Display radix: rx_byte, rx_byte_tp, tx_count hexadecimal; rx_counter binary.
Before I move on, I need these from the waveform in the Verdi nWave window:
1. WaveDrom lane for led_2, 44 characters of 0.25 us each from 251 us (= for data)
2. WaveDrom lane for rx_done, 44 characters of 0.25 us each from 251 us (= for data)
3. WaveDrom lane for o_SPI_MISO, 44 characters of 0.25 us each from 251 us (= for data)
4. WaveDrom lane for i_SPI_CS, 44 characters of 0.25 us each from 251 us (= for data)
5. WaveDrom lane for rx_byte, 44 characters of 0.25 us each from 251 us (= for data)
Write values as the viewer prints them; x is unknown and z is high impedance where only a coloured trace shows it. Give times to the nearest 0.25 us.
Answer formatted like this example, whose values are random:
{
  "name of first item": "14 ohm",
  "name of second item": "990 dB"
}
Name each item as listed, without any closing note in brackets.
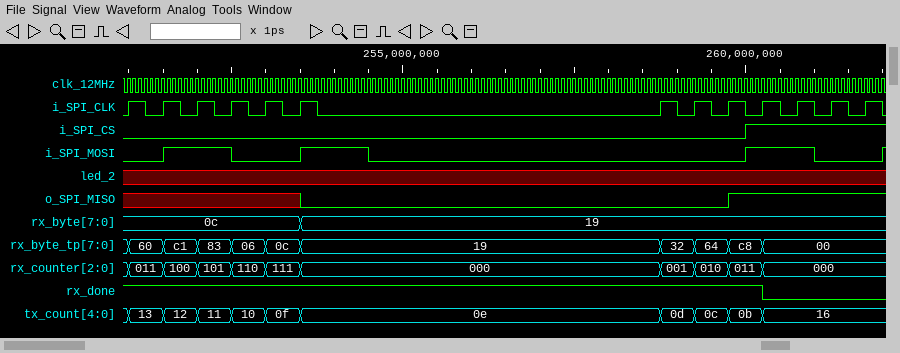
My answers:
{
  "WaveDrom lane for led_2, 44 characters of 0.25 us each from 251 us": "{name: 'led_2', wave: 'x...........................................'}",
  "WaveDrom lane for rx_done, 44 characters of 0.25 us each from 251 us": "{name: 'rx_done', wave: '1....................................0......'}",
  "WaveDrom lane for o_SPI_MISO, 44 characters of 0.25 us each from 251 us": "{name: 'o_SPI_MISO', wave: 'x.........0........................1........'}",
  "WaveDrom lane for i_SPI_CS, 44 characters of 0.25 us each from 251 us": "{name: 'i_SPI_CS', wave: '0...................................1.......'}",
  "WaveDrom lane for rx_byte, 44 characters of 0.25 us each from 251 us": "{name: 'rx_byte', wave: '=.........=.................................', data: '0c 19'}"
}
